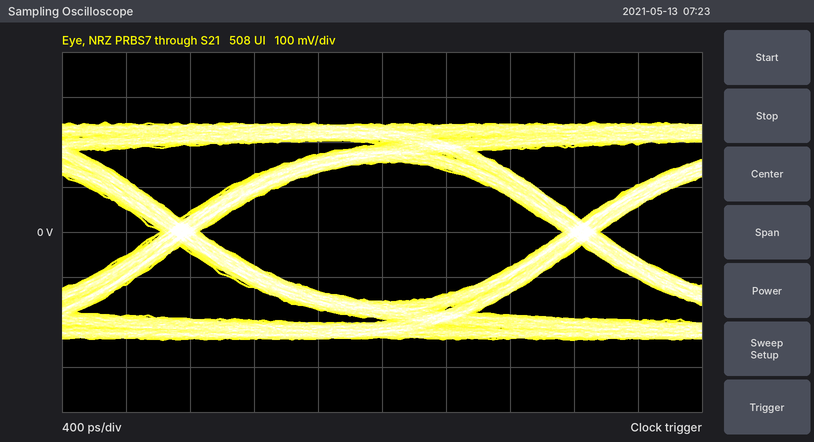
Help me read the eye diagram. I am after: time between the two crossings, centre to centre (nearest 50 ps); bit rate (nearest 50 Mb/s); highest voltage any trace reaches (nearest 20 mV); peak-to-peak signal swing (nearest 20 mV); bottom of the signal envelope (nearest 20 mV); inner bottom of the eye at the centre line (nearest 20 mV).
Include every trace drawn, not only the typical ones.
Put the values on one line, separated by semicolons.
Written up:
2.50 ns; 400 Mb/s; 240 mV; 480 mV; -240 mV; -160 mV
